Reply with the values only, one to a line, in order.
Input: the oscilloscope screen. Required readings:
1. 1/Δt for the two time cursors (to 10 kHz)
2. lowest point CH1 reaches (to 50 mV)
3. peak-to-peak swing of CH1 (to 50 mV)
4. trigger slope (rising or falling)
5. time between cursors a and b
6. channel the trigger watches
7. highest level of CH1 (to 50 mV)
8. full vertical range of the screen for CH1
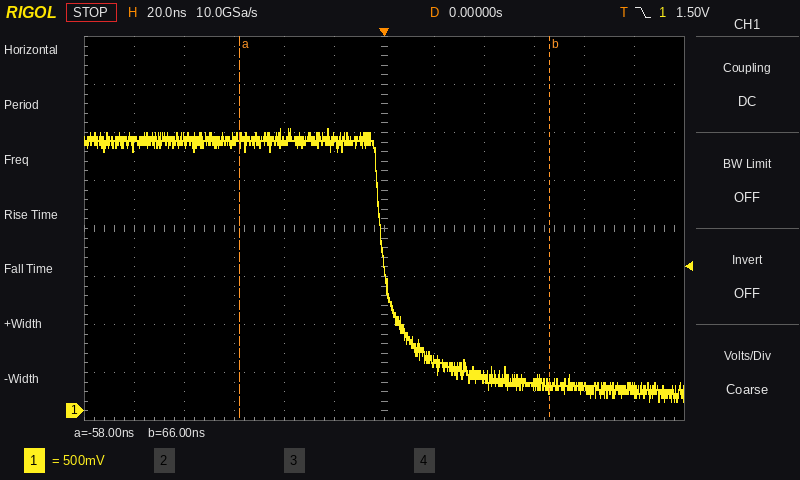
8.06 MHz
100 mV
2.85 V
falling
124 ns
CH1
2.95 V
4 V
